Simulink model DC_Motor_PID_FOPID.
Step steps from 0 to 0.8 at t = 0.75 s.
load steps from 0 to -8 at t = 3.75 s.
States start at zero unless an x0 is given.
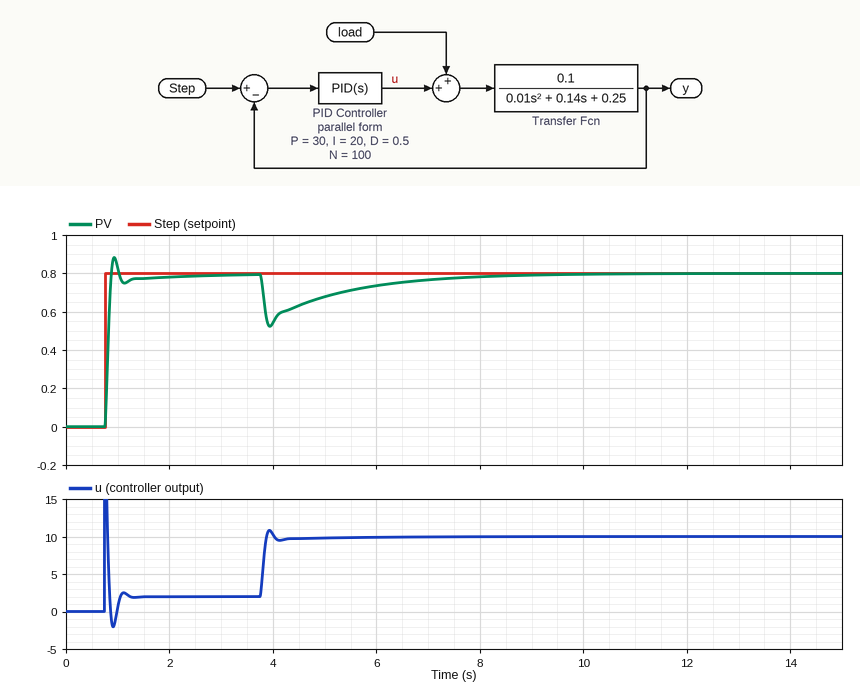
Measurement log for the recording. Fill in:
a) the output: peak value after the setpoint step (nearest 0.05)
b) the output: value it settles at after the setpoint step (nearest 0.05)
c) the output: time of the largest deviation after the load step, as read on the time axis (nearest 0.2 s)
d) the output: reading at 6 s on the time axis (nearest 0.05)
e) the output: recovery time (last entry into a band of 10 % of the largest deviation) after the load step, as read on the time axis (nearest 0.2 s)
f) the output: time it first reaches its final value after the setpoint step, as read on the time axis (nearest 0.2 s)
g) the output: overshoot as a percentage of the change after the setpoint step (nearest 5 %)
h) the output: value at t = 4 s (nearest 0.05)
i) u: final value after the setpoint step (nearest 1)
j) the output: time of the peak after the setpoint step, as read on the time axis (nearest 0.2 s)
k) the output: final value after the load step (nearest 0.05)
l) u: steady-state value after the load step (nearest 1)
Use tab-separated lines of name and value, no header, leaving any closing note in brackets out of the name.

the output: peak value after the setpoint step	0.90
the output: value it settles at after the setpoint step	0.80
the output: time of the largest deviation after the load step, as read on the time axis	4.0 s
the output: reading at 6 s on the time axis	0.75
the output: recovery time (last entry into a band of 10 % of the largest deviation) after the load step, as read on the time axis	7.4 s
the output: time it first reaches its final value after the setpoint step, as read on the time axis	0.8 s
the output: overshoot as a percentage of the change after the setpoint step	10 %
the output: value at t = 4 s	0.55
u: final value after the setpoint step	2
the output: time of the peak after the setpoint step, as read on the time axis	1.0 s
the output: final value after the load step	0.80
u: steady-state value after the load step	10
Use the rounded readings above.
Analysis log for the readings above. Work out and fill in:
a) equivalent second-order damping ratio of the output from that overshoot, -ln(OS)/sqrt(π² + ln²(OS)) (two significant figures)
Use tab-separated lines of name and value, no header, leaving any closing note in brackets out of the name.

equivalent second-order damping ratio of the output from that overshoot, -ln(OS)/sqrt(π² + ln²(OS))	0.59
